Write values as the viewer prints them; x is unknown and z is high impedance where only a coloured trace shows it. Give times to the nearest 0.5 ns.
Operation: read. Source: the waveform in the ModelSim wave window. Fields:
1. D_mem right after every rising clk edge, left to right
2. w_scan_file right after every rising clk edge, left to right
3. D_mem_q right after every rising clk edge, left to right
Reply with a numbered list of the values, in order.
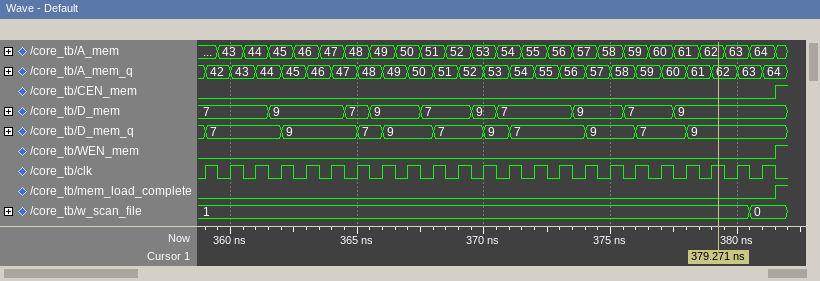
1. 7, 7, 7, 9, 9, 9, 7, 9, 9, 7, 7, 9, 7, 7, 7, 9, 9, 7, 7, 9, 9, 9, 9
2. 1, 1, 1, 1, 1, 1, 1, 1, 1, 1, 1, 1, 1, 1, 1, 1, 1, 1, 1, 1, 1, 1, 0
3. 7, 7, 7, 9, 9, 9, 7, 9, 9, 7, 7, 9, 7, 7, 7, 9, 9, 7, 7, 9, 9, 9, 9
